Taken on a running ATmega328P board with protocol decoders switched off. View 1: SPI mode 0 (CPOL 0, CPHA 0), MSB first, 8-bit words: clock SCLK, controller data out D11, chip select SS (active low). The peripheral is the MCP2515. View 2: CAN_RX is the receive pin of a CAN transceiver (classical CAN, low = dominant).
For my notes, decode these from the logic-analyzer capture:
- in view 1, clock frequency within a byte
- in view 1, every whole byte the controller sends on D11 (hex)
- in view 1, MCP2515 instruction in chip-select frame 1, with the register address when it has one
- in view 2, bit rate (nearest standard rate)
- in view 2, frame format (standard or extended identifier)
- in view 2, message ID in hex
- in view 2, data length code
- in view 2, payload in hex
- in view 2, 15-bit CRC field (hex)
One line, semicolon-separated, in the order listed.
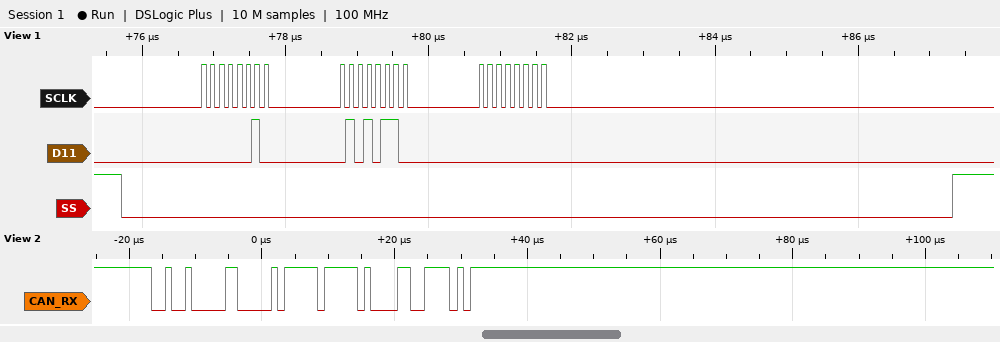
8 MHz; 0x02 0x56 0x00; WRITE 0x56; 1000 kbit/s; standard; 0x241; 1; FF; 0x619E
